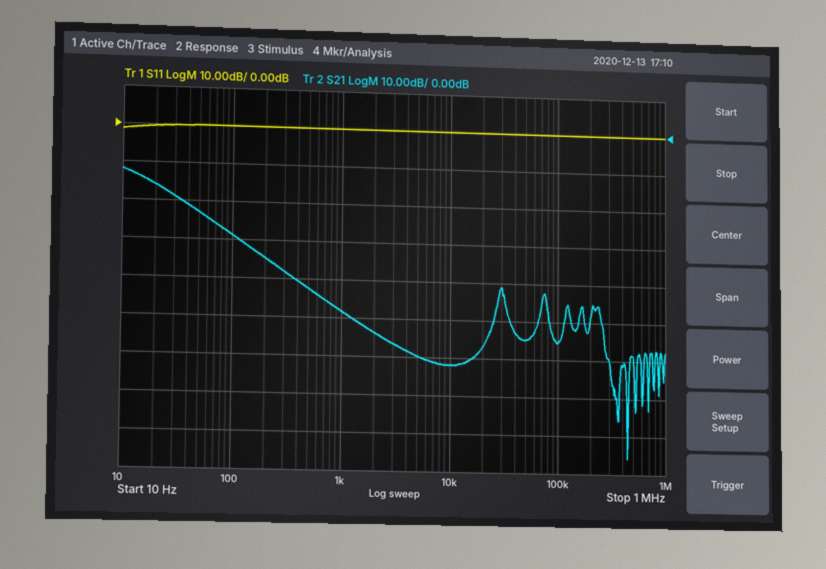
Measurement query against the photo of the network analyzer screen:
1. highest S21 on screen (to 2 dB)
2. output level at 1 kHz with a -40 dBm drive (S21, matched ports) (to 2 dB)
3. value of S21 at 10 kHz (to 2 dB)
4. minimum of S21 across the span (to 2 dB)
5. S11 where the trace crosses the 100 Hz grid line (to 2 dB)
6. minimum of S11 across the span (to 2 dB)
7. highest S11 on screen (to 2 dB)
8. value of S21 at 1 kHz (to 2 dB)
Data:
-12 dB
-88 dBm
-62 dB
-86 dB
0 dB
-2 dB
0 dB
-48 dB
